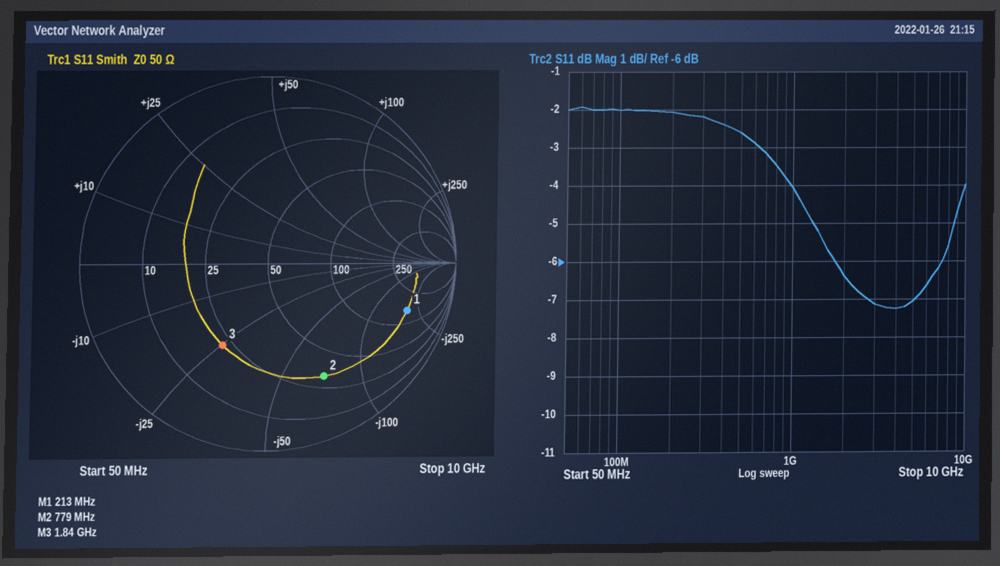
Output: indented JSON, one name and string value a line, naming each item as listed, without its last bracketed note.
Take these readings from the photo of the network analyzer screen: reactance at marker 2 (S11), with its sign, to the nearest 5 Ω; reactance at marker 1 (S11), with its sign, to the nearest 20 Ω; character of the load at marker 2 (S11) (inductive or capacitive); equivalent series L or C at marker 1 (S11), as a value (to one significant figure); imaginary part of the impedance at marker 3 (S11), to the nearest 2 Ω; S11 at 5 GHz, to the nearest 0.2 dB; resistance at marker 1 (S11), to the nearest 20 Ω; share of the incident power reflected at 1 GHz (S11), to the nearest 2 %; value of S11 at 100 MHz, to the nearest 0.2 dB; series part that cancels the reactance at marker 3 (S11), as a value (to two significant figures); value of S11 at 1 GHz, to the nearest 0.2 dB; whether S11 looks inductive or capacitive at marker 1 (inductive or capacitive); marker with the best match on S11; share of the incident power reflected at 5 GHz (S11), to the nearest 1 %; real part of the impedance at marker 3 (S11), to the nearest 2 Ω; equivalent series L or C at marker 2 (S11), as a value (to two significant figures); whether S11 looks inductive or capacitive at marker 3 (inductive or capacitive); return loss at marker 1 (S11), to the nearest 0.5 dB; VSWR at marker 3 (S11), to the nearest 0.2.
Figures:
{
  "reactance at marker 2 (S11), with its sign, to the nearest 5 Ω": "-70 Ω",
  "reactance at marker 1 (S11), with its sign, to the nearest 20 Ω": "-200 Ω",
  "character of the load at marker 2 (S11)": "capacitive",
  "equivalent series L or C at marker 1 (S11), as a value": "4 pF",
  "imaginary part of the impedance at marker 3 (S11), to the nearest 2 Ω": "-26 Ω",
  "S11 at 5 GHz, to the nearest 0.2 dB": "-7.0 dB",
  "resistance at marker 1 (S11), to the nearest 20 Ω": "140 Ω",
  "share of the incident power reflected at 1 GHz (S11), to the nearest 2 %": "40 %",
  "value of S11 at 100 MHz, to the nearest 0.2 dB": "-2.0 dB",
  "series part that cancels the reactance at marker 3 (S11), as a value": "2.2 nH",
  "value of S11 at 1 GHz, to the nearest 0.2 dB": "-4.0 dB",
  "whether S11 looks inductive or capacitive at marker 1": "capacitive",
  "marker with the best match on S11": "marker 3",
  "share of the incident power reflected at 5 GHz (S11), to the nearest 1 %": "20 %",
  "real part of the impedance at marker 3 (S11), to the nearest 2 Ω": "22 Ω",
  "equivalent series L or C at marker 2 (S11), as a value": "2.9 pF",
  "whether S11 looks inductive or capacitive at marker 3": "capacitive",
  "return loss at marker 1 (S11), to the nearest 0.5 dB": "2.0 dB",
  "VSWR at marker 3 (S11), to the nearest 0.2": "3.0"
}
